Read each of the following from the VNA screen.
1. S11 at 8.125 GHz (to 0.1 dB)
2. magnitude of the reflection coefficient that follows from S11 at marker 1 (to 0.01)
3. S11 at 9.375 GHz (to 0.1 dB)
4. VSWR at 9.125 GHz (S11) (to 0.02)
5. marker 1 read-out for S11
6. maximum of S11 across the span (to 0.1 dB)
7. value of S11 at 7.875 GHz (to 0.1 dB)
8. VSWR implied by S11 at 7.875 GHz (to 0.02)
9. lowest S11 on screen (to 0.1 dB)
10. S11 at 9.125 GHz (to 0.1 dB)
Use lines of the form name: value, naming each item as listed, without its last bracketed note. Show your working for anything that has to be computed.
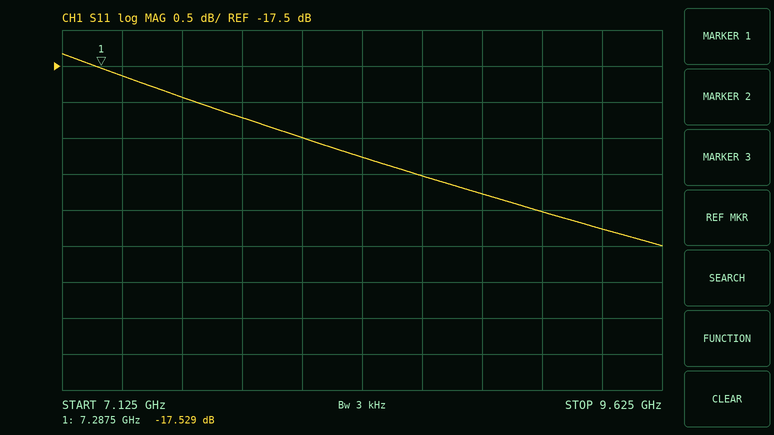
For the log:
S11 at 8.125 GHz: -18.5 dB
magnitude of the reflection coefficient that follows from S11 at marker 1: 10^(-17.529/20) ≈ 0.13
S11 at 9.375 GHz: -19.8 dB
VSWR at 9.125 GHz (S11): |Γ| = 10^(-19.5/20) = 0.1059; VSWR = (1 + 0.1059)/(1 − 0.1059) ≈ 1.24
marker 1 read-out for S11: -17.529 dB
maximum of S11 across the span: -17.3 dB
value of S11 at 7.875 GHz: -18.2 dB
VSWR implied by S11 at 7.875 GHz: |Γ| = 10^(-18.2/20) = 0.1230; VSWR = (1 + 0.1230)/(1 − 0.1230) ≈ 1.28
lowest S11 on screen: -20.0 dB
S11 at 9.125 GHz: -19.5 dB
